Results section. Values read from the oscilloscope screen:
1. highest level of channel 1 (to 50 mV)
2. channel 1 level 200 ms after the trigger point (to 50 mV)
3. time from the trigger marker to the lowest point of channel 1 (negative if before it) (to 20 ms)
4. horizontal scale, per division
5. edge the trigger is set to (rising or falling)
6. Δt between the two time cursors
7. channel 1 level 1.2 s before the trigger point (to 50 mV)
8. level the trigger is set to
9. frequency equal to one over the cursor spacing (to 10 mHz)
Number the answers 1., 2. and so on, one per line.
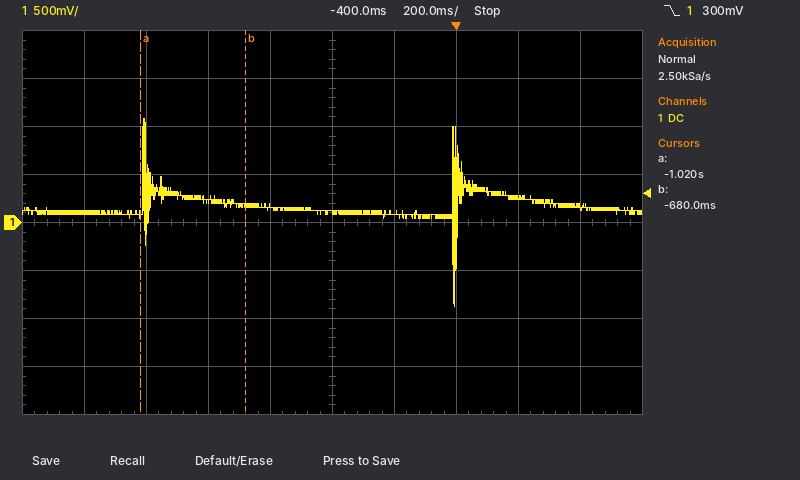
1. 1.10 V
2. 250 mV
3. 0 ms
4. 200 ms
5. falling
6. 340 ms
7. 100 mV
8. 300 mV
9. 2.94 Hz
